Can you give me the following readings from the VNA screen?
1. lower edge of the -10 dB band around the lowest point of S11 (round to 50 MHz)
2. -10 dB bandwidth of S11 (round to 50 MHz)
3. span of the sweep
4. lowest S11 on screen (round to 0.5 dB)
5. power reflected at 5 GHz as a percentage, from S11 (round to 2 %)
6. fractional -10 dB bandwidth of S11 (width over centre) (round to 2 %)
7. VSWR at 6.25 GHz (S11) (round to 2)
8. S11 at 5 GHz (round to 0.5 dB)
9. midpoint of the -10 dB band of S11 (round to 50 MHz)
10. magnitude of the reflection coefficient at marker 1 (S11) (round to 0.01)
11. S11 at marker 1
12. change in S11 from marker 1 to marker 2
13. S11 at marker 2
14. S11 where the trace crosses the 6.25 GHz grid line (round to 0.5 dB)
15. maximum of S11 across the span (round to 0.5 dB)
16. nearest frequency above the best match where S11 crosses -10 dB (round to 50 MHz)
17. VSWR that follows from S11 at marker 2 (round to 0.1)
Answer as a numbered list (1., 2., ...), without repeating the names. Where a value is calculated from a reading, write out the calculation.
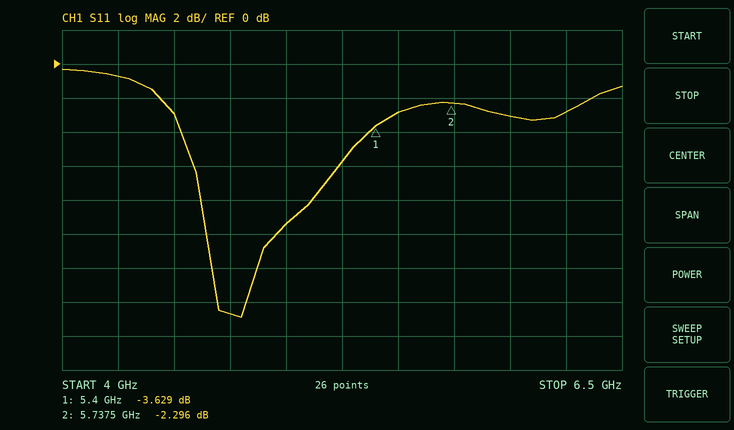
1. 4.65 GHz
2. 4.95 GHz − 4.65 GHz = 300 MHz
3. 2.5 GHz
4. -15.0 dB
5. 10^(-9.5/10) ≈ 11.2 %, so 12 % to the nearest 2 %
6. 300 MHz / 4.8 GHz ≈ 6 %
7. |Γ| = 10^(-3/20) = 0.7079; VSWR = (1 + 0.7079)/(1 − 0.7079) ≈ 6
8. -9.5 dB
9. 4.80 GHz
10. 10^(-3.629/20) ≈ 0.66
11. -3.629 dB
12. -2.296 − (-3.629) = 1.333 dB
13. -2.296 dB
14. -3.0 dB
15. -0.5 dB
16. 4.95 GHz
17. (1 + 0.7677)/(1 − 0.7677) ≈ 7.6
